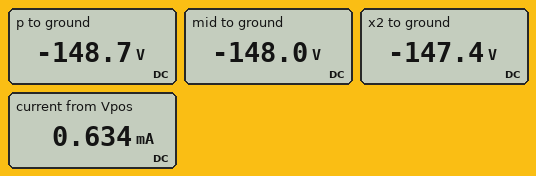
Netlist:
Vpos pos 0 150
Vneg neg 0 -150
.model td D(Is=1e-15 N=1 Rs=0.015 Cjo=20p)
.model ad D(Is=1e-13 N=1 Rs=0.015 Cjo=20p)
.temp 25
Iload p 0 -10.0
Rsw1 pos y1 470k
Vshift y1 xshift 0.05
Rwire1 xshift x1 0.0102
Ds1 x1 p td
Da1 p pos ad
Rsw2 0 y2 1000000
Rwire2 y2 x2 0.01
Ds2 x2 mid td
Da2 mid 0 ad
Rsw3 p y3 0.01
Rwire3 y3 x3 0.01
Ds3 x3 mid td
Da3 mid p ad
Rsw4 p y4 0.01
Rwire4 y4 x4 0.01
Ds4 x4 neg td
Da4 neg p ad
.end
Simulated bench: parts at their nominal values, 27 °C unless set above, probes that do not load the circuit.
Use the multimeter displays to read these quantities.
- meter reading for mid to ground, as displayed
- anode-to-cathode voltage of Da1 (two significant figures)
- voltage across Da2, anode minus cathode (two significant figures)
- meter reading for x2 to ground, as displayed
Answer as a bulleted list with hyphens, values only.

- -148.0 V
- -300 V
- -150 V
- -147.4 V
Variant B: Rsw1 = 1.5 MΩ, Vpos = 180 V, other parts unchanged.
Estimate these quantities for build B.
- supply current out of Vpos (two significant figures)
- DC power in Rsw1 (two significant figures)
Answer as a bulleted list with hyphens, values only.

- 220 µA
- 72 mW
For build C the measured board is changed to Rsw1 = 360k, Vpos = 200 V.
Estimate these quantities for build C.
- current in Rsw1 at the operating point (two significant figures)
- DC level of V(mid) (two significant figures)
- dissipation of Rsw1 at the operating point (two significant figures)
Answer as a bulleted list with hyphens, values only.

- 970 µA
- -150 V
- 340 mW
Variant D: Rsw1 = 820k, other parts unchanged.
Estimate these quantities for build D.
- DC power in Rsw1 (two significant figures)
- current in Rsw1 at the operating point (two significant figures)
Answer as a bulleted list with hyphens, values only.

- 110 mW
- 360 µA
